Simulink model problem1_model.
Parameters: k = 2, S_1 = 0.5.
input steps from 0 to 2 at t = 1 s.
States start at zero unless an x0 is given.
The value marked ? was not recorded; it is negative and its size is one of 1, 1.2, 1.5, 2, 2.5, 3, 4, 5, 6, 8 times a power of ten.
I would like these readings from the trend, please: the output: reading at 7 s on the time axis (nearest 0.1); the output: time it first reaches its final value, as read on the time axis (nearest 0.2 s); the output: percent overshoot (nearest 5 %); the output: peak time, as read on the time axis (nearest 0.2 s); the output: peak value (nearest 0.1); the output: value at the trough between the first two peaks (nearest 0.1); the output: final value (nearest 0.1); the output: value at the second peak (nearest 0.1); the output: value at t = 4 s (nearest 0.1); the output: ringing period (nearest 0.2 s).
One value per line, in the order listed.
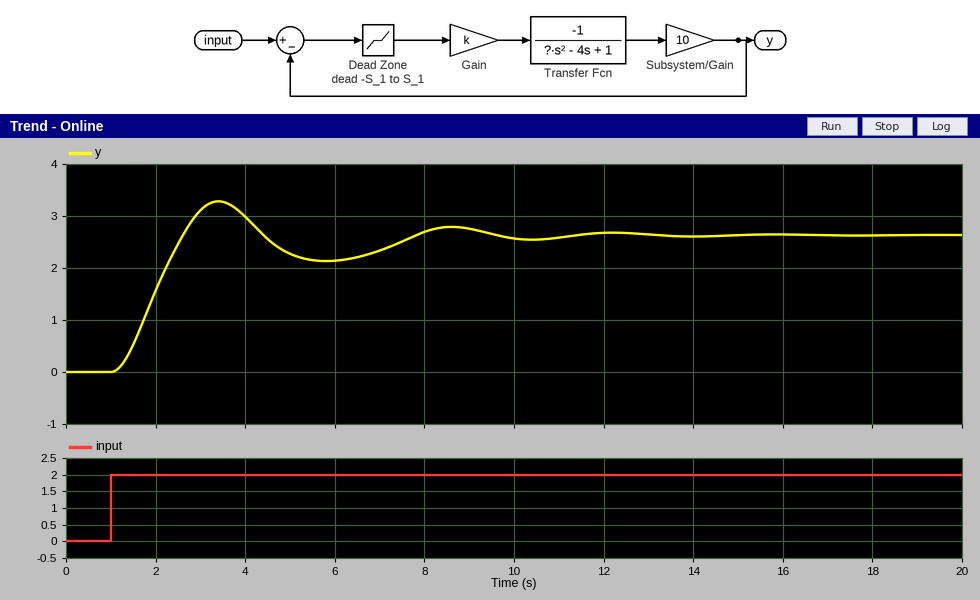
2.3
2.6 s
25 %
3.4 s
3.3
2.1
2.6
2.8
3.0
5.2 s
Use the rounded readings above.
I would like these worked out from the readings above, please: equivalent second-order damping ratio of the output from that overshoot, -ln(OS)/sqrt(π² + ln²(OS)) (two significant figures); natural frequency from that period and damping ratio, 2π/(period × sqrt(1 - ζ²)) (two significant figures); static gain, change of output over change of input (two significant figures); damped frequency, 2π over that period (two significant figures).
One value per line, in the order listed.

0.40
1.3 rad/s
1.3
1.2 rad/s
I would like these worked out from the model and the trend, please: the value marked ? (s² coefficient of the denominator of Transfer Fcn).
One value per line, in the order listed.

-6
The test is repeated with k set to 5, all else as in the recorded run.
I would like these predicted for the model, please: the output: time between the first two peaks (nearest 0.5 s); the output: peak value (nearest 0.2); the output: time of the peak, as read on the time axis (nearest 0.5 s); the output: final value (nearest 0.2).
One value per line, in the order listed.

4.5 s
3.4
2.5 s
2.6
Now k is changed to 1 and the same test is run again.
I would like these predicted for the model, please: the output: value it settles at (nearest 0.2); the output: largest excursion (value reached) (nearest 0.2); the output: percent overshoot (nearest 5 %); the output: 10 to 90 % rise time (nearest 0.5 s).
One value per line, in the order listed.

2.8
3.2
15 %
2.0 s
